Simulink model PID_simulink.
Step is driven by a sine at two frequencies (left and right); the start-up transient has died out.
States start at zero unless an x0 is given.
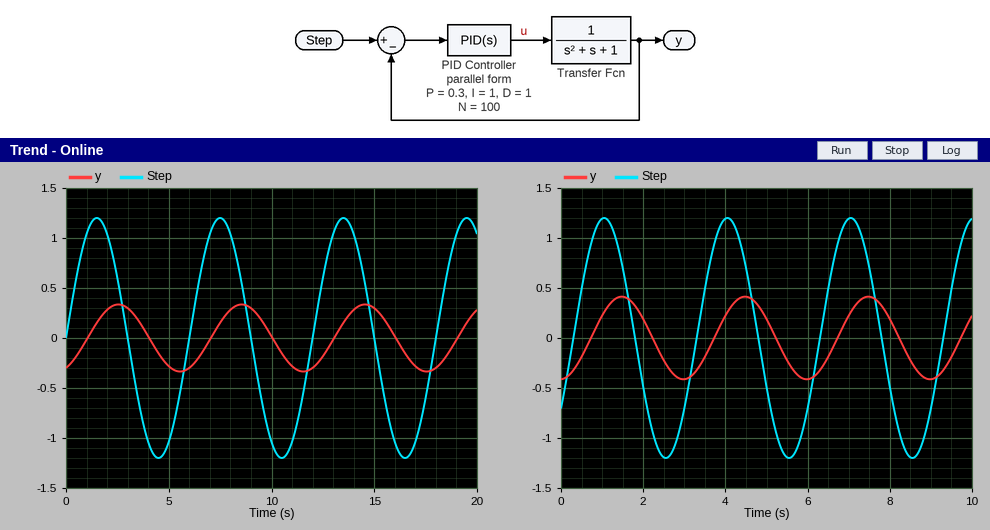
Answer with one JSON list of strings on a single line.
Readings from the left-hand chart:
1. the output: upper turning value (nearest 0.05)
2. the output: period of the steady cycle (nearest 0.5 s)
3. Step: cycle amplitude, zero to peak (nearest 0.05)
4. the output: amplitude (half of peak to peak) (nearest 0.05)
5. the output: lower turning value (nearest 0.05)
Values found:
["0.35", "6.0 s", "1.20", "0.35", "-0.35"]
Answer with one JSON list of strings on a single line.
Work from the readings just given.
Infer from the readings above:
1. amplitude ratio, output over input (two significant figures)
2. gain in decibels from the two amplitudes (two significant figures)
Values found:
["0.29", "-11 dB"]
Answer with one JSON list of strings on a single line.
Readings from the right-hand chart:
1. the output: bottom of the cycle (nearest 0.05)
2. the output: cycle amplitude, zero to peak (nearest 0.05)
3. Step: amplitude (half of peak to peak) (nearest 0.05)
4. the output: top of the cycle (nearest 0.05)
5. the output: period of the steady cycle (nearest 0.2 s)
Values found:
["-0.40", "0.40", "1.20", "0.40", "3.0 s"]
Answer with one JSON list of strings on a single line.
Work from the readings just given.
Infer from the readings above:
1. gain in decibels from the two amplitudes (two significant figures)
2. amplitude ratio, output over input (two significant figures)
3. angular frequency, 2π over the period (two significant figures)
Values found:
["-9.5 dB", "0.33", "2.1 rad/s"]
